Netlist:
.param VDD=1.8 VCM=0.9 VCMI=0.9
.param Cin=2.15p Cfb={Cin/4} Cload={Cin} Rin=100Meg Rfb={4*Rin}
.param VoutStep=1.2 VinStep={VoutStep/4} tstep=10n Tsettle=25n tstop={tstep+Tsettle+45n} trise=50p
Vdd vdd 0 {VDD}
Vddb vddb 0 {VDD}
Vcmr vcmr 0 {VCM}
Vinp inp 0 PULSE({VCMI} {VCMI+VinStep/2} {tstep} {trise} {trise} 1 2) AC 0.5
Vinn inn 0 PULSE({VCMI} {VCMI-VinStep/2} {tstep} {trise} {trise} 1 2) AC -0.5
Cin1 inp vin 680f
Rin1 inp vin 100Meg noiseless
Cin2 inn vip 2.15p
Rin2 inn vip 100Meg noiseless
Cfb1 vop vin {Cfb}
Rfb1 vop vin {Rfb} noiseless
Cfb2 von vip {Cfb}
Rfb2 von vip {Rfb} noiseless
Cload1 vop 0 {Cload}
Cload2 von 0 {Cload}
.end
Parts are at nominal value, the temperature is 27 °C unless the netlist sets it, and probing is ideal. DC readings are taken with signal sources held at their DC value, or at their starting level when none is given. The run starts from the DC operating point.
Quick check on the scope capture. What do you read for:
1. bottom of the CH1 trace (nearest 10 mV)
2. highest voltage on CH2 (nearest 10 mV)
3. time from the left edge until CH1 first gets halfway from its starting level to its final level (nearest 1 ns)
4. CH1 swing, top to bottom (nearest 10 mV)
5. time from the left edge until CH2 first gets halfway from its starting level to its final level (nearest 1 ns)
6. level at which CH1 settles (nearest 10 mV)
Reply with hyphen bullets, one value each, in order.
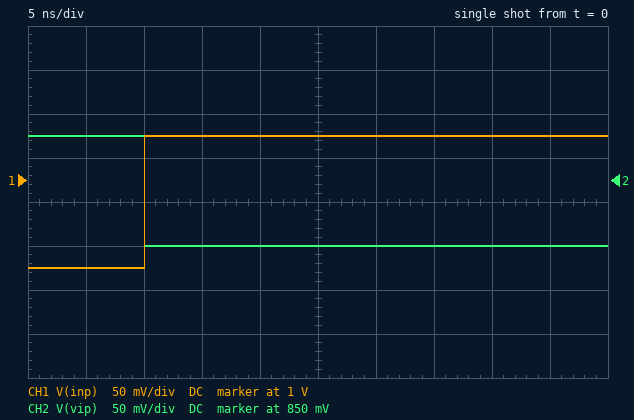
- 900 mV
- 900 mV
- 10 ns
- 150 mV
- 10 ns
- 1.05 V
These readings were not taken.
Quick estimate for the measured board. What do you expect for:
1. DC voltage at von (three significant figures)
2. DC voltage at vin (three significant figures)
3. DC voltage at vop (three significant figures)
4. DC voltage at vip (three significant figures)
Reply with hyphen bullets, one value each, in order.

- 900 mV
- 900 mV
- 900 mV
- 900 mV
